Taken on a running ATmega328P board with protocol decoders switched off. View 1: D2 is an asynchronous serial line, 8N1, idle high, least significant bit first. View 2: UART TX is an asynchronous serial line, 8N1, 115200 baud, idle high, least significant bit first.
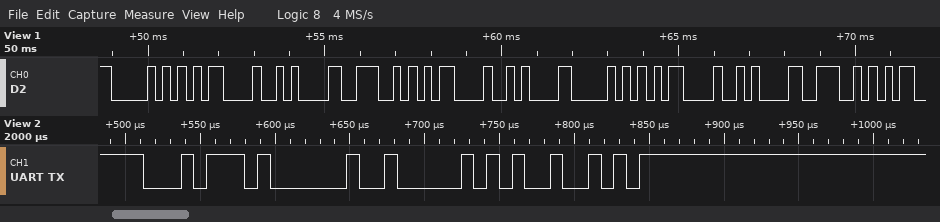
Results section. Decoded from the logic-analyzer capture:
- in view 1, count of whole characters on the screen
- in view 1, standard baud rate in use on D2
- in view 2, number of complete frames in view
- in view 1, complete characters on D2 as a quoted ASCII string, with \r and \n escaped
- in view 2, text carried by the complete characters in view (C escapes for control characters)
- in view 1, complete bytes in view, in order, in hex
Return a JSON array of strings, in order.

["10", "4800 baud", "4", "\"P\\r\\nN\\r\\nP\\r\\nN\"", "\"t PR\"", "0x50 0x0D 0x0A 0x4E 0x0D 0x0A 0x50 0x0D 0x0A 0x4E"]
